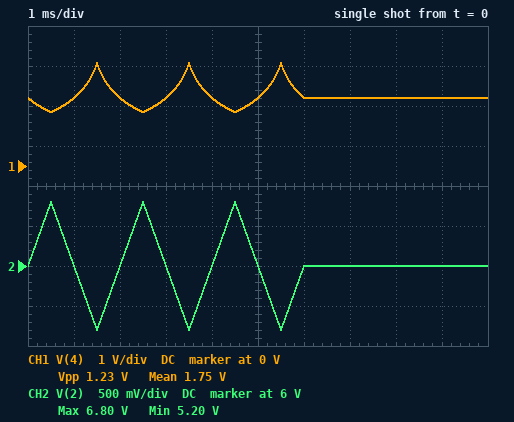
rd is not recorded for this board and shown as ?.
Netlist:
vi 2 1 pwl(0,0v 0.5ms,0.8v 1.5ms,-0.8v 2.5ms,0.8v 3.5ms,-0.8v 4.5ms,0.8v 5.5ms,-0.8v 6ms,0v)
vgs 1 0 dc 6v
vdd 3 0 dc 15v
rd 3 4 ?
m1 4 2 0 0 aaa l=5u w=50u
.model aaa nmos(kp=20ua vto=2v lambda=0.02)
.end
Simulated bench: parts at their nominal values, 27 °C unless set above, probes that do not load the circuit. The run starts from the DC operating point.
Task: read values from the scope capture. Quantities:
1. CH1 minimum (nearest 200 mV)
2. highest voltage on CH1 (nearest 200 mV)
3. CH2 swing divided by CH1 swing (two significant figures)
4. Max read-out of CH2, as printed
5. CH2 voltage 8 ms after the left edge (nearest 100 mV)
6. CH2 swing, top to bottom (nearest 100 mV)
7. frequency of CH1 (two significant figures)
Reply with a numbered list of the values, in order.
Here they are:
1. 1.4 V
2. 2.6 V
3. 1.3
4. 6.80 V
5. 6.0 V
6. 1.6 V
7. 500 Hz
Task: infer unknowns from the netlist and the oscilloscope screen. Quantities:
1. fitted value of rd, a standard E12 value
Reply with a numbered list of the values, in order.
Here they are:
1. 12 kΩ
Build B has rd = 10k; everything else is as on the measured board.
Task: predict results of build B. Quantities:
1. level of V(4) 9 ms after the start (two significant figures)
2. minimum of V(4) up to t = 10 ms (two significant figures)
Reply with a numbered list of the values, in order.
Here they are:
1. 2.1 V
2. 1.6 V
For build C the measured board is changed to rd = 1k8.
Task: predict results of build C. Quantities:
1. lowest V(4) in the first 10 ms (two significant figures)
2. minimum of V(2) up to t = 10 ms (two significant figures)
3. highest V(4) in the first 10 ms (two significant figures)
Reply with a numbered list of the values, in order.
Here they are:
1. 10 V
2. 5.2 V
3. 13 V
